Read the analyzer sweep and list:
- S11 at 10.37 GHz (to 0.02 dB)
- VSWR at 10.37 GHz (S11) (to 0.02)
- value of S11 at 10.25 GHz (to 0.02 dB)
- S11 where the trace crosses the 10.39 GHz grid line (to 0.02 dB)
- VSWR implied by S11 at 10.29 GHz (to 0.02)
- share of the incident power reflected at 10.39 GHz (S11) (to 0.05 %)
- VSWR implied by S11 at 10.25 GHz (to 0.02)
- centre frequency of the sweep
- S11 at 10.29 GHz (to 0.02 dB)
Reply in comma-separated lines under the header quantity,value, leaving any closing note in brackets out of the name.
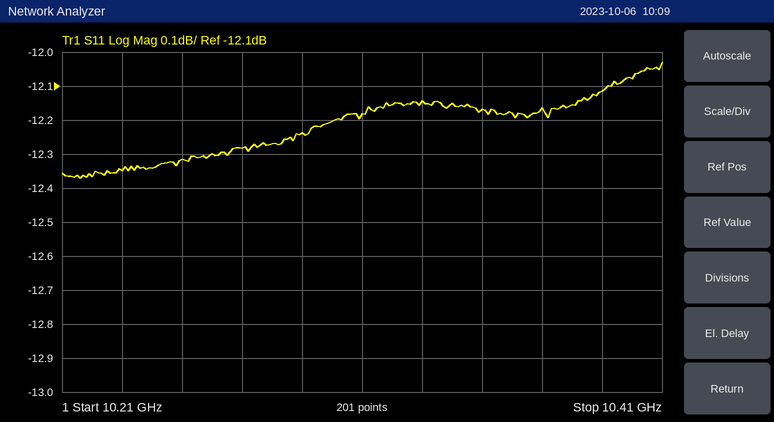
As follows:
quantity,value
S11 at 10.37 GHz,-12.16 dB
VSWR at 10.37 GHz (S11),1.66
value of S11 at 10.25 GHz,-12.32 dB
S11 where the trace crosses the 10.39 GHz grid line,-12.12 dB
VSWR implied by S11 at 10.29 GHz,1.64
share of the incident power reflected at 10.39 GHz (S11),6.15 %
VSWR implied by S11 at 10.25 GHz,1.64
centre frequency of the sweep,10.31 GHz
S11 at 10.29 GHz,-12.24 dB
